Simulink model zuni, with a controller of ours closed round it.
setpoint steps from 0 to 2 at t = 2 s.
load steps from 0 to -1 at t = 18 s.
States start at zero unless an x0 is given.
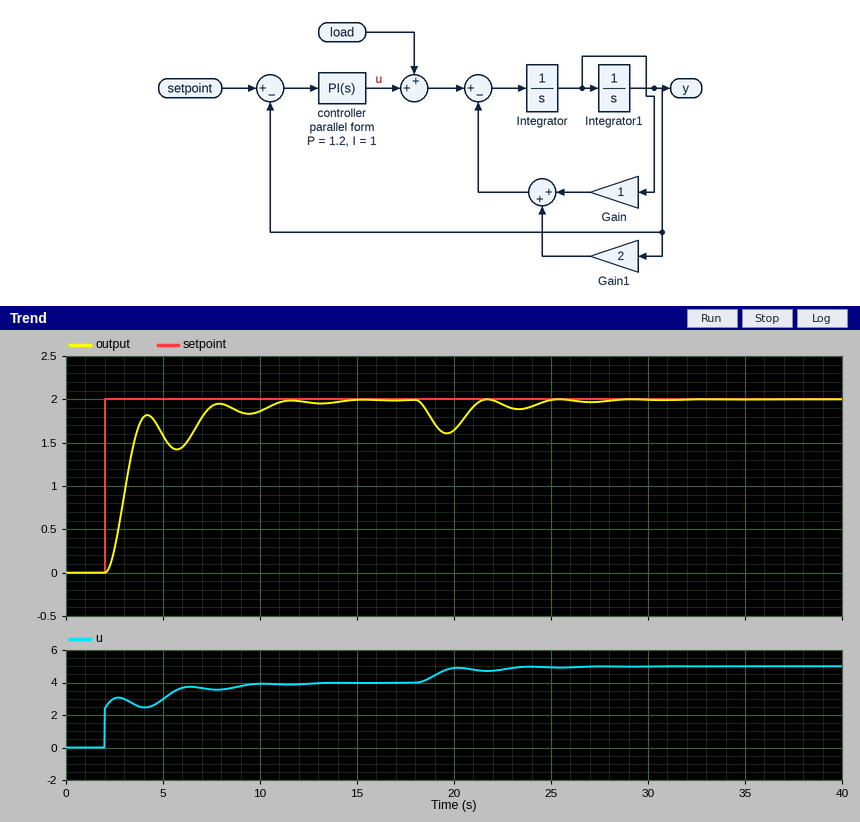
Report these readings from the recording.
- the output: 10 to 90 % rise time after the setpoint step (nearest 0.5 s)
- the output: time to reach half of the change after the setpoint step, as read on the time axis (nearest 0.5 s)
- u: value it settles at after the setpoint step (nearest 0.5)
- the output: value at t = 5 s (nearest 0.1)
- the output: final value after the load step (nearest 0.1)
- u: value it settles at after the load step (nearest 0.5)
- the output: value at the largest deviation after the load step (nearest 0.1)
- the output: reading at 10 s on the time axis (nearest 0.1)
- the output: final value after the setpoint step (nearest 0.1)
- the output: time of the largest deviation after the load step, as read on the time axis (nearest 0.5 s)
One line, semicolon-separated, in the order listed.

1.5 s; 3.0 s; 4.0; 1.6; 2.0; 5.0; 1.6; 1.9; 2.0; 19.5 s
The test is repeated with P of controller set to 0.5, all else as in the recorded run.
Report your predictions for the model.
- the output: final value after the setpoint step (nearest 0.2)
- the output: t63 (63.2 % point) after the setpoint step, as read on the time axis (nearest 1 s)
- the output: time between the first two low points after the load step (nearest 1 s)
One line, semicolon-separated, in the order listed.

2.0; 4 s; 4 s
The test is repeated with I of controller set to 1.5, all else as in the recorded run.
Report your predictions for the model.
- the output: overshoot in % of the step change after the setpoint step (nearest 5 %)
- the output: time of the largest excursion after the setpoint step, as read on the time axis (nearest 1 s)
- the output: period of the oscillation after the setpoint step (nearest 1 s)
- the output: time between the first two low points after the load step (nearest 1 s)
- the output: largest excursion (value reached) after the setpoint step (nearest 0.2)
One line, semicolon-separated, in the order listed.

10 %; 8 s; 4 s; 4 s; 2.2
